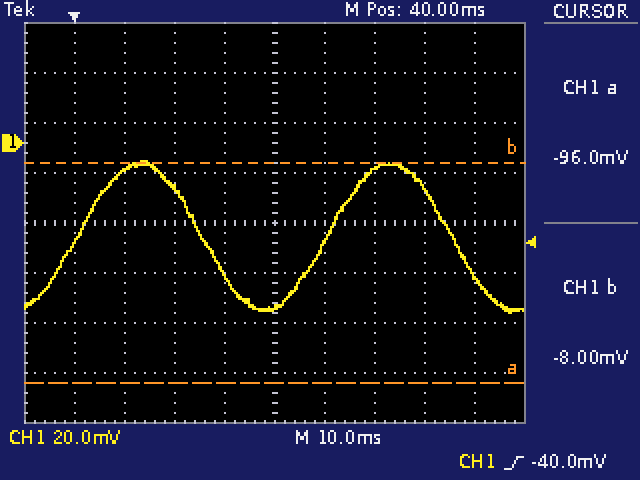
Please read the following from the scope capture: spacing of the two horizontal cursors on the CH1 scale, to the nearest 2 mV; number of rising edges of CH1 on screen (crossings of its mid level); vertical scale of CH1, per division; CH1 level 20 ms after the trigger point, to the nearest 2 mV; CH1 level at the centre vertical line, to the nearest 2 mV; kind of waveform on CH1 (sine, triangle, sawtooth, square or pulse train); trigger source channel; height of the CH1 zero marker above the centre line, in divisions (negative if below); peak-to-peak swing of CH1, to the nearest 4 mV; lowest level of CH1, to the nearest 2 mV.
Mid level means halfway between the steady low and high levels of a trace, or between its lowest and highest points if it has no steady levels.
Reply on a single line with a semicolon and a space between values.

88 mV; 2; 20 mV; -18 mV; -66 mV; sine; CH1; +1.6 div; 60 mV; -68 mV
